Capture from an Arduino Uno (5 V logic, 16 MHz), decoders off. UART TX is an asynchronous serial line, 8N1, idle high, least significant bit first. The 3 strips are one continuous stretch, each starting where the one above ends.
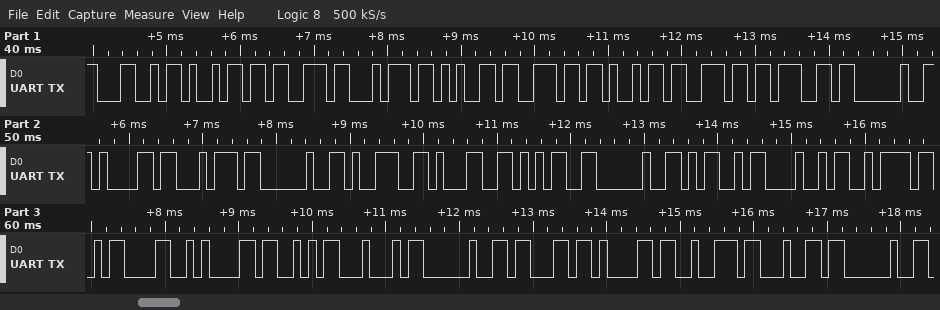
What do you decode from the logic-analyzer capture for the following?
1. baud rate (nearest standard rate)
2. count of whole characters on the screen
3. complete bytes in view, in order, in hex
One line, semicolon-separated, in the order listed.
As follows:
9600 baud; 30; 4C 69 73 74 65 6E 69 6E 67 20 61 74 20 39 31 35 20 4D 48 7A 0D 0A 53 44 20 63 61 72 64 20
